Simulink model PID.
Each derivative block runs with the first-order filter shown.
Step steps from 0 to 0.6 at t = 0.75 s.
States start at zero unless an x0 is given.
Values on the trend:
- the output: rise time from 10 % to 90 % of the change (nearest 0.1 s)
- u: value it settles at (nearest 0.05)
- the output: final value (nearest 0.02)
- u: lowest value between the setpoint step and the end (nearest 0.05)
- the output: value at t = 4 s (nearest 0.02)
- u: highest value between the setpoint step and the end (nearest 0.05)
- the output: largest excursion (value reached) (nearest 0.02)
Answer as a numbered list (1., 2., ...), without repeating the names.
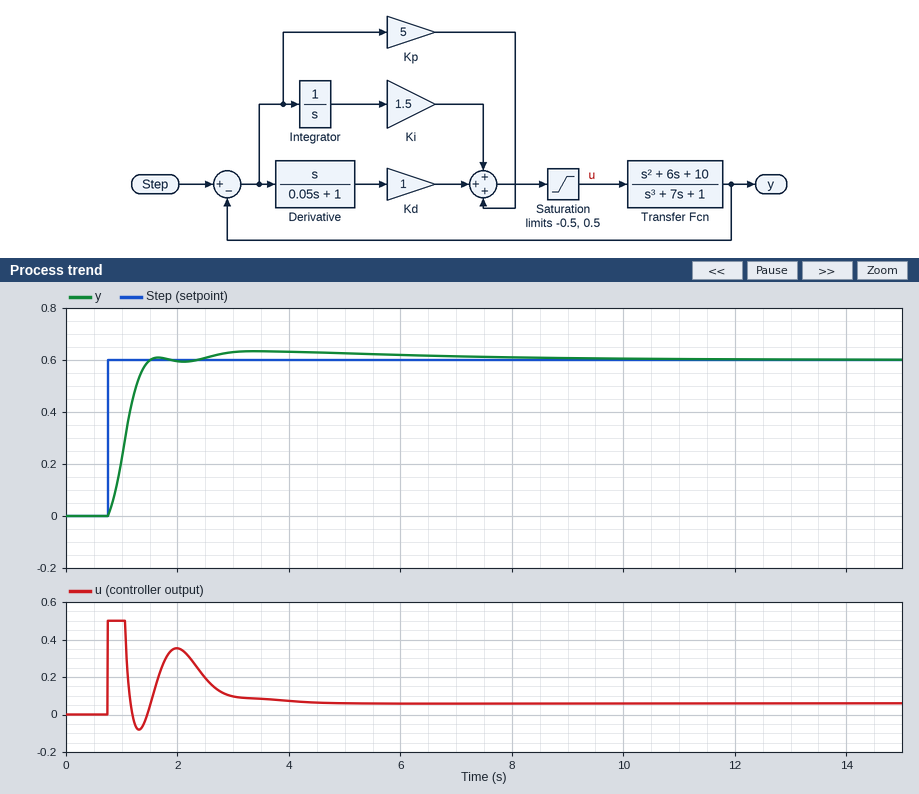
1. 0.5 s
2. 0.05
3. 0.60
4. -0.10
5. 0.64
6. 0.50
7. 0.64
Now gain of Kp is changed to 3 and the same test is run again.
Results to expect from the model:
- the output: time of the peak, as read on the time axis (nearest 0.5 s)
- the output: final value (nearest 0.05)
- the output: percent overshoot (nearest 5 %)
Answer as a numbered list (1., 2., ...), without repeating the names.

1. 3.5 s
2. 0.60
3. 10 %
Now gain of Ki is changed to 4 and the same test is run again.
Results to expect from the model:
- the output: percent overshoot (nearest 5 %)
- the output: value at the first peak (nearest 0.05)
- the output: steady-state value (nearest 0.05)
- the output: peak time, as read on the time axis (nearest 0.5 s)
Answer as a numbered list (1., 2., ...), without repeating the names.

1. 15 %
2. 0.70
3. 0.60
4. 1.5 s
